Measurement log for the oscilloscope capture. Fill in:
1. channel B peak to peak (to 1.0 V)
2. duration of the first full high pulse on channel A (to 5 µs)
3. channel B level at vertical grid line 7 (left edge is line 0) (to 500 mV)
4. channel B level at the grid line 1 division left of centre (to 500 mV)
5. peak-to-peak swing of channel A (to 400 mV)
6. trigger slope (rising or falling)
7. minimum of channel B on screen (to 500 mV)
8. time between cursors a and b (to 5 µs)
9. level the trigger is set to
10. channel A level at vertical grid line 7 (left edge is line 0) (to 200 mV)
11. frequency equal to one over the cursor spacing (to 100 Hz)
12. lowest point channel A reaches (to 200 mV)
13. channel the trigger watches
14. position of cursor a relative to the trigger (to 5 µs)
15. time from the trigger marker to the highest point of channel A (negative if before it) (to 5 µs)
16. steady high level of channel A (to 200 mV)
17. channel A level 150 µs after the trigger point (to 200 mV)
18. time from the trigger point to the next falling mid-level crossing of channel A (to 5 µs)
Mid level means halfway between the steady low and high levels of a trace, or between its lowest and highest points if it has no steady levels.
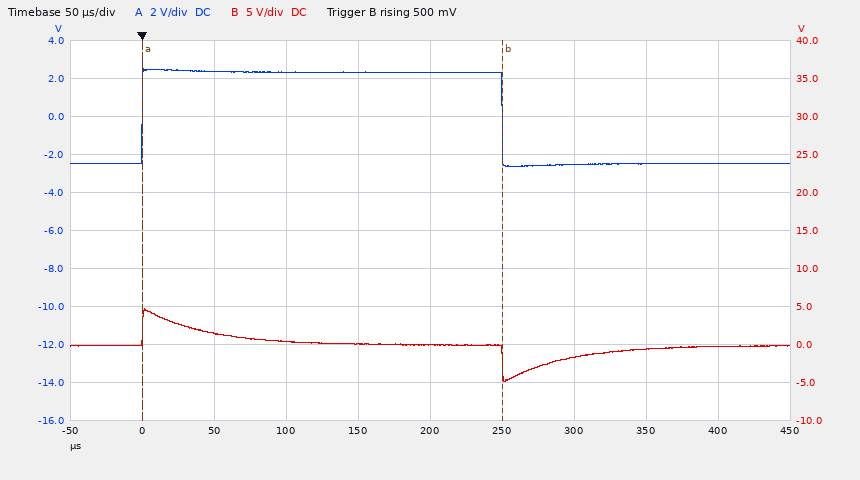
10.0 V
250 µs
-1.5 V
0.0 V
5.6 V
rising
-5.0 V
250 µs
500 mV
-2.6 V
4.0 kHz
-2.6 V
channel B
0 µs
0 µs
2.4 V
2.4 V
250 µs
